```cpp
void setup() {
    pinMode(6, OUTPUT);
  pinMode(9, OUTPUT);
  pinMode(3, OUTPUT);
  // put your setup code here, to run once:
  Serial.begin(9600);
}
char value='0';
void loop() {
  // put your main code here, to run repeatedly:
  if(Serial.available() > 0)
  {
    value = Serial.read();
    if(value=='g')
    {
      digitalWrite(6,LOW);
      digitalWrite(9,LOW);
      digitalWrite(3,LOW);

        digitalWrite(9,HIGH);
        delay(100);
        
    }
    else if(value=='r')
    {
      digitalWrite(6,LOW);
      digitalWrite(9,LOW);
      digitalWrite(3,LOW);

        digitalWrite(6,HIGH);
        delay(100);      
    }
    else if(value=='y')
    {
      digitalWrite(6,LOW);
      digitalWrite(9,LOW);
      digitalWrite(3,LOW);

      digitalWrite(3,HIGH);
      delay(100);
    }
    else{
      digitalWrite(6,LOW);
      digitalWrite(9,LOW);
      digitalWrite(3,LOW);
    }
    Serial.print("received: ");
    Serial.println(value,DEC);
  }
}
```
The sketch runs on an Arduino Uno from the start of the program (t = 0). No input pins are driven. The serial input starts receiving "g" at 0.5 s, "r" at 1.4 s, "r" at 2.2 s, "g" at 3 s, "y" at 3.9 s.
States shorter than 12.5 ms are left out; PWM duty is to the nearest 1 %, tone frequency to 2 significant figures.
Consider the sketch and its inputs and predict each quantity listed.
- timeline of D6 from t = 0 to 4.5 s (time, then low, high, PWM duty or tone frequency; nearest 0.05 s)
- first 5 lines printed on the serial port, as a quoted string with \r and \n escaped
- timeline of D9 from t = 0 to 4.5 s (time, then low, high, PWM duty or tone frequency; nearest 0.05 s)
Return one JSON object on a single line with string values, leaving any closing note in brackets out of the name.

{"timeline of D6 from t = 0 to 4.5 s": "0 s low; 1.4 s high; 3 s low", "first 5 lines printed on the serial port, as a quoted string with \\r and \\n escaped": "\"received: 103\\r\\nreceived: 114\\r\\nreceived: 114\\r\\nreceived: 103\\r\\nreceived: 121\\r\\n\"", "timeline of D9 from t = 0 to 4.5 s": "0 s low; 0.5 s high; 1.4 s low; 3 s high; 3.9 s low"}
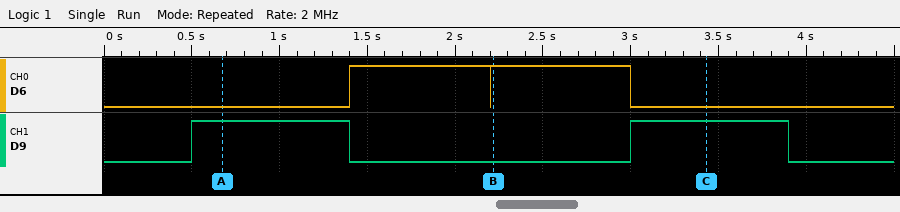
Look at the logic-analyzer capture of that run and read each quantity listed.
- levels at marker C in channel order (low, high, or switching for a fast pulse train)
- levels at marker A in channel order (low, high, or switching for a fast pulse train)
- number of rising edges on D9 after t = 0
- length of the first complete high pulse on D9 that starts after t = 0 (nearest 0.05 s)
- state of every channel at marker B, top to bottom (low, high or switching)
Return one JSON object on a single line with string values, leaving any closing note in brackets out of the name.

{"levels at marker C in channel order": "D6 low, D9 high", "levels at marker A in channel order": "D6 low, D9 high", "number of rising edges on D9 after t = 0": "2", "length of the first complete high pulse on D9 that starts after t = 0": "0.90 s", "state of every channel at marker B, top to bottom": "D6 high, D9 low"}
